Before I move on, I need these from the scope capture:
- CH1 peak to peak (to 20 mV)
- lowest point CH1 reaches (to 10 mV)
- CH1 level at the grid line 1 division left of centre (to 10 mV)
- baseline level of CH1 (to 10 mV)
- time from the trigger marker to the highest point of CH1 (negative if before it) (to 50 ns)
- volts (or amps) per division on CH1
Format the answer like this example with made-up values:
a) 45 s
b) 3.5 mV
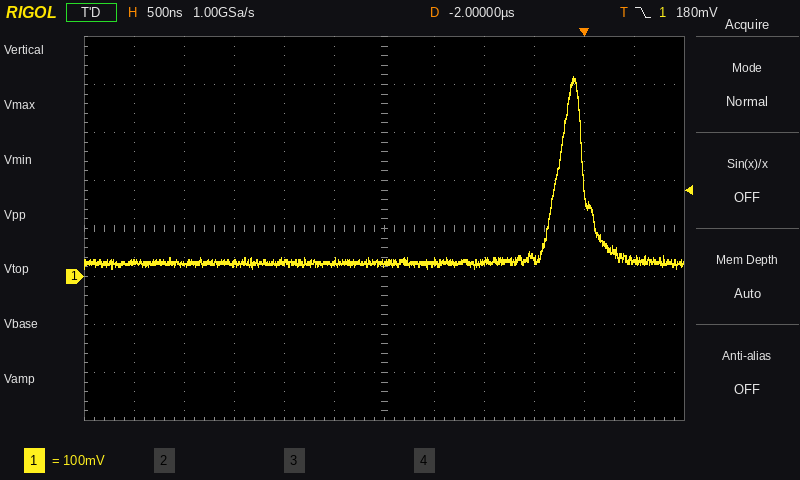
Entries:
a) 400 mV
b) 20 mV
c) 30 mV
d) 30 mV
e) -100 ns
f) 100 mV
